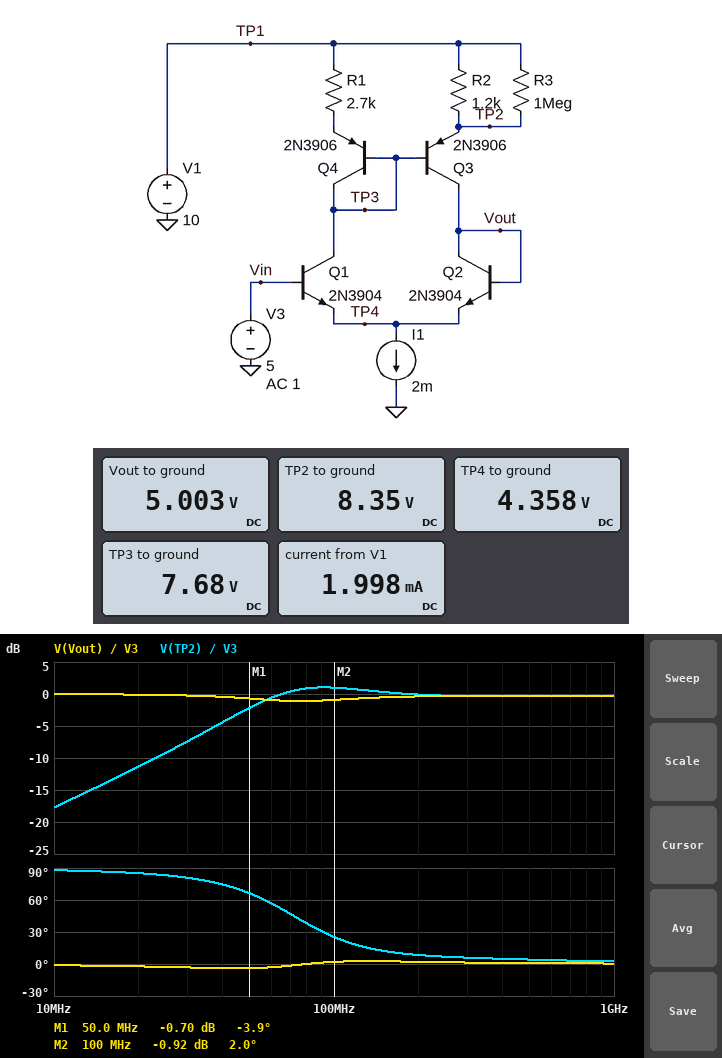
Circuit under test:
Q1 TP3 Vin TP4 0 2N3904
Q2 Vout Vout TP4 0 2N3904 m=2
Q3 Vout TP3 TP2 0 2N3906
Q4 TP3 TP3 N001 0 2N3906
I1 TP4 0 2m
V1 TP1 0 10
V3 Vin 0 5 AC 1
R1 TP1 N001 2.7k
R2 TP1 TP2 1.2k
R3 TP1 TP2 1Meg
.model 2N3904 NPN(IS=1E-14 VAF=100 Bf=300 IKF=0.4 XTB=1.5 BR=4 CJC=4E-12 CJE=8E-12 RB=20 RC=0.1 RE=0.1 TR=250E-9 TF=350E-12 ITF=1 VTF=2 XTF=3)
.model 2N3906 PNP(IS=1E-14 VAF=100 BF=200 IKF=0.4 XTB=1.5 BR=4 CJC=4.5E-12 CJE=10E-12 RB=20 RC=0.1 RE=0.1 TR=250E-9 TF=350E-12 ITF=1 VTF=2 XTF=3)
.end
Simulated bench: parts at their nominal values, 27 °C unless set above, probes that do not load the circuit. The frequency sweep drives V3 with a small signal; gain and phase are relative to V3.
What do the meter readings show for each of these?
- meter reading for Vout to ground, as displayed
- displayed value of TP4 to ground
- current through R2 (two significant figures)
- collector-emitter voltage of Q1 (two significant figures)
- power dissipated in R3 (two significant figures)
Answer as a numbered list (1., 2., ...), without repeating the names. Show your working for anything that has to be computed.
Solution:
1. 5.003 V
2. 4.358 V
3. (10 V - 8.35 V) / 1.2 kΩ = 1.4 mA
4. 7.68 V - 4.358 V = 3.3 V
5. (10 V - 8.35 V)^2 / 1 MΩ = 2.7 µW
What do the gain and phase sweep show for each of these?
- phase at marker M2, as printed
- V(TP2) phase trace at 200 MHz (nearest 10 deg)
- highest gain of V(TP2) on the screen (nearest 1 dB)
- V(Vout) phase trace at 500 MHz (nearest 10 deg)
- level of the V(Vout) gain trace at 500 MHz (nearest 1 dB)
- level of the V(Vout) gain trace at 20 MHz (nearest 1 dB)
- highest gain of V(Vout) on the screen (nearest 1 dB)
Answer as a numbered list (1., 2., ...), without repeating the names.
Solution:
1. 2.0 deg
2. 10 deg
3. 1 dB
4. 0 deg
5. 0 dB
6. 0 dB
7. 0 dB
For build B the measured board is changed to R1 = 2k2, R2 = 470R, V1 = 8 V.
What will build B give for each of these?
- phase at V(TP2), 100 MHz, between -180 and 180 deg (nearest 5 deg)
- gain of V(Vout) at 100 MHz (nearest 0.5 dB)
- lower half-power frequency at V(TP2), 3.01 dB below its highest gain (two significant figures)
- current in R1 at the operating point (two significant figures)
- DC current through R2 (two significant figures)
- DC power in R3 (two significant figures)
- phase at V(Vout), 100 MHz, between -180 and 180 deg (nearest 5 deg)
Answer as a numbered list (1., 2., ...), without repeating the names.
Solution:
1. 35 deg
2. -2.5 dB
3. 62 MHz
4. 370 µA
5. 1.6 mA
6. 590 nW
7. 5 deg
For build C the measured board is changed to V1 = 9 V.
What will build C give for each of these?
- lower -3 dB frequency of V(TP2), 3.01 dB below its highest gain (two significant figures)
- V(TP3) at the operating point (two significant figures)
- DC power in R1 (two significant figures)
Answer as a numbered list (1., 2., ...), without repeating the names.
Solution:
1. 47 MHz
2. 6.7 V
3. 1.0 mW
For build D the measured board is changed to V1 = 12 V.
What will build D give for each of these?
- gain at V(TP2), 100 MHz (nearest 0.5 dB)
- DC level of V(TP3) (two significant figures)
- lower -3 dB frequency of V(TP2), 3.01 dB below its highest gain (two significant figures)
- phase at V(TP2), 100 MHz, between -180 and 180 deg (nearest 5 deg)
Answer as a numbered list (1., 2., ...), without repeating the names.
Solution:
1. 1.0 dB
2. 9.7 V
3. 56 MHz
4. 30 deg
